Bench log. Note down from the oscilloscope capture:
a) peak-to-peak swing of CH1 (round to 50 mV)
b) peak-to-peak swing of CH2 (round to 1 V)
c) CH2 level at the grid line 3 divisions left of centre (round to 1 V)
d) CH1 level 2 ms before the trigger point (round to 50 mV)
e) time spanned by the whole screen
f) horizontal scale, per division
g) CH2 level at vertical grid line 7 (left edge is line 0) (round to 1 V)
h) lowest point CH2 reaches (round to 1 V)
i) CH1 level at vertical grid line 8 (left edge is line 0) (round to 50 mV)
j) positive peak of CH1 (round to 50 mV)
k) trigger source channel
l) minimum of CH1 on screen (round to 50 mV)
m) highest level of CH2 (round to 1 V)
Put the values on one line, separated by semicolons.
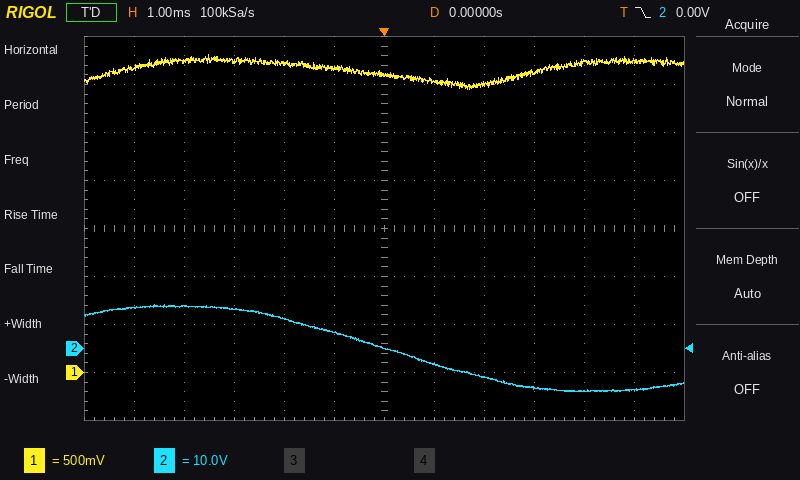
350 mV; 18 V; 8 V; 3.20 V; 12 ms; 1 ms; -3 V; -9 V; 3.00 V; 3.30 V; CH2; 2.95 V; 9 V
